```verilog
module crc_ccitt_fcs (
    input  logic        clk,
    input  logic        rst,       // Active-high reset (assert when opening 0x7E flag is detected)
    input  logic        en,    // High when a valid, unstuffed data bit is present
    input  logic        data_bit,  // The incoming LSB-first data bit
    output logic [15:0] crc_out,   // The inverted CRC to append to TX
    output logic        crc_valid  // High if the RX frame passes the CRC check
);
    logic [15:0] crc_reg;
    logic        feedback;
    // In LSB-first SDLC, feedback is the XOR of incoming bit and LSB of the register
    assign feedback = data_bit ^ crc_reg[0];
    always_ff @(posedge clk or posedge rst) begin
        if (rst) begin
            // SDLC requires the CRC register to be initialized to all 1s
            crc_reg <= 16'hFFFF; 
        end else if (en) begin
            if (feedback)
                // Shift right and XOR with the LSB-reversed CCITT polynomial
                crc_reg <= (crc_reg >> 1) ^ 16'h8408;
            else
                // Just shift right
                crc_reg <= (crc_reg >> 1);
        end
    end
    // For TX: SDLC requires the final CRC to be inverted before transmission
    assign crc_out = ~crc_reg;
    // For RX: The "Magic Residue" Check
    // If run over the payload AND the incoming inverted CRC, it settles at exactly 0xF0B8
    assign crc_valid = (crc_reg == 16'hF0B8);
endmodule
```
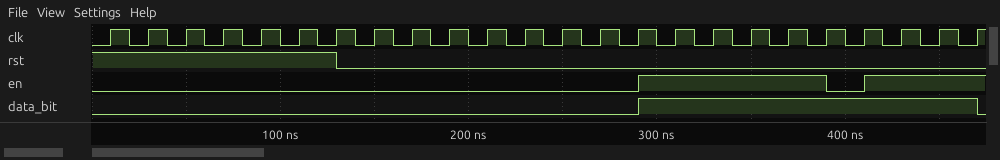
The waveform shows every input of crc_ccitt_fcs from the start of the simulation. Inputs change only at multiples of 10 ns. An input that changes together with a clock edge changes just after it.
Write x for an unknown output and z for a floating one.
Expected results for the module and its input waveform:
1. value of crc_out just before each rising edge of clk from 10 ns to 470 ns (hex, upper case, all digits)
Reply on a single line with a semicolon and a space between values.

0000, 0000, 0000, 0000, 0000, 0000, 0000, 0000, 0000, 0000, 0000, 0000, 0000, 0000, 0000, 0000, 8000, C000, E000, F000, F800, F800, FC00, FE00
